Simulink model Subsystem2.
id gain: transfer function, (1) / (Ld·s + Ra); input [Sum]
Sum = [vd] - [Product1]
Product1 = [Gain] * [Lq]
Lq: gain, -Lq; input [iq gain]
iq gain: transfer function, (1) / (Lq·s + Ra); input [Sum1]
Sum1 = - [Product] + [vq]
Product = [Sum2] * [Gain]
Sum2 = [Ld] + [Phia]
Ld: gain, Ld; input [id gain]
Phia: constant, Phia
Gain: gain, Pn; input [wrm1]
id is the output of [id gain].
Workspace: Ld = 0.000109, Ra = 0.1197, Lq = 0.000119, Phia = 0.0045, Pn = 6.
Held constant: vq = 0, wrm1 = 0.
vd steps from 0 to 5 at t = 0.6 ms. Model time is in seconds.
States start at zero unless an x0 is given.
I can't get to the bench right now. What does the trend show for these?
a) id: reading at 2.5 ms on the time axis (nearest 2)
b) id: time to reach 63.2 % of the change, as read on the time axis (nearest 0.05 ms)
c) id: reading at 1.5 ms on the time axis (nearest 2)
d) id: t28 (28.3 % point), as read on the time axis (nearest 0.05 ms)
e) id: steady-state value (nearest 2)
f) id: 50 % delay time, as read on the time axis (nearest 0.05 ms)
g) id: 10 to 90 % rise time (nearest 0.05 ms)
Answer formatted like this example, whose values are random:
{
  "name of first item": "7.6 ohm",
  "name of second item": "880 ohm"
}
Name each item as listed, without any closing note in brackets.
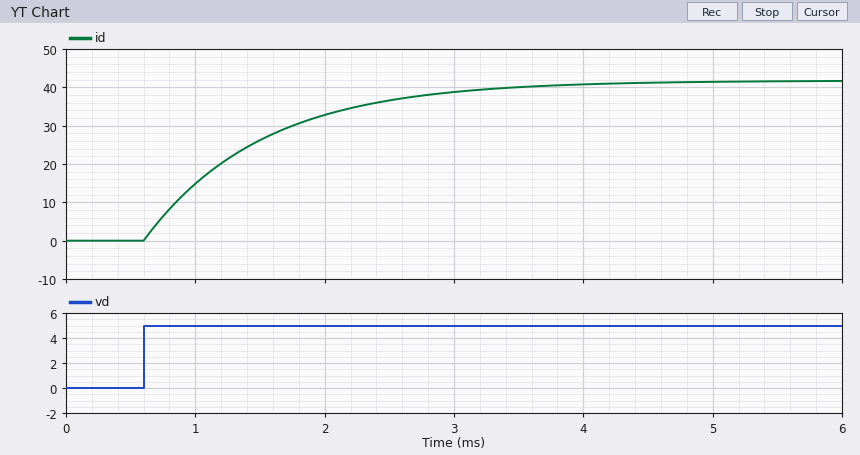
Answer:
{
  "id: reading at 2.5 ms on the time axis": "36",
  "id: time to reach 63.2 % of the change, as read on the time axis": "1.50 ms",
  "id: reading at 1.5 ms on the time axis": "26",
  "id: t28 (28.3 % point), as read on the time axis": "0.90 ms",
  "id: steady-state value": "42",
  "id: 50 % delay time, as read on the time axis": "1.25 ms",
  "id: 10 to 90 % rise time": "2.00 ms"
}
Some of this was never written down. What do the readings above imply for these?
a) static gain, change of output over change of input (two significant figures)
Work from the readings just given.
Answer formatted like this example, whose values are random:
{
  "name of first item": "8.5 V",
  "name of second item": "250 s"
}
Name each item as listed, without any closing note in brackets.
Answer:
{
  "static gain, change of output over change of input": "8.4"
}
